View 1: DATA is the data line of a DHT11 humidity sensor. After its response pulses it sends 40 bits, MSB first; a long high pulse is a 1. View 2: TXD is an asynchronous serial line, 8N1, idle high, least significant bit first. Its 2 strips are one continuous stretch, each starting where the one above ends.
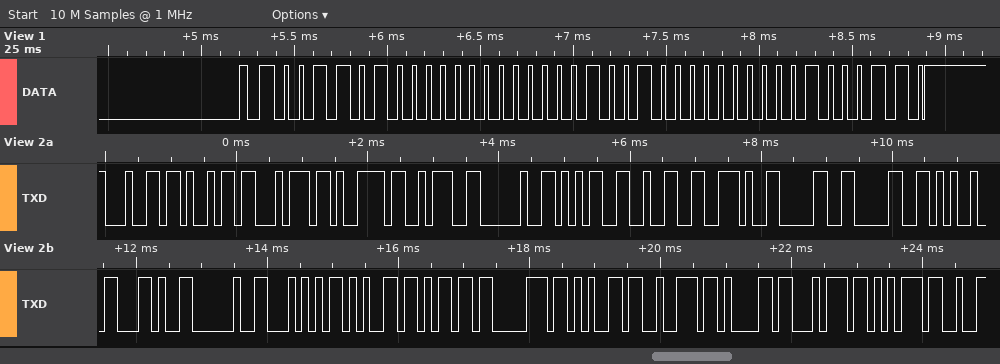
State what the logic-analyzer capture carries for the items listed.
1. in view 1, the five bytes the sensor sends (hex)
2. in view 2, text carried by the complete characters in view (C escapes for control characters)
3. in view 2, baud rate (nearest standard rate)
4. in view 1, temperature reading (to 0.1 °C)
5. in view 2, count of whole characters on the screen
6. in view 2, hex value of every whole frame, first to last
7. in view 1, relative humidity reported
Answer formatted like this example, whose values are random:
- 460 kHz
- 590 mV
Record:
- 34 00 12 00 46
- "dity: 52.00%, Temperatu"
- 9600 baud
- 18.0 °C
- 23
- 0x64 0x69 0x74 0x79 0x3A 0x20 0x35 0x32 0x2E 0x30 0x30 0x25 0x2C 0x20 0x54 0x65 0x6D 0x70 0x65 0x72 0x61 0x74 0x75
- 52 %
